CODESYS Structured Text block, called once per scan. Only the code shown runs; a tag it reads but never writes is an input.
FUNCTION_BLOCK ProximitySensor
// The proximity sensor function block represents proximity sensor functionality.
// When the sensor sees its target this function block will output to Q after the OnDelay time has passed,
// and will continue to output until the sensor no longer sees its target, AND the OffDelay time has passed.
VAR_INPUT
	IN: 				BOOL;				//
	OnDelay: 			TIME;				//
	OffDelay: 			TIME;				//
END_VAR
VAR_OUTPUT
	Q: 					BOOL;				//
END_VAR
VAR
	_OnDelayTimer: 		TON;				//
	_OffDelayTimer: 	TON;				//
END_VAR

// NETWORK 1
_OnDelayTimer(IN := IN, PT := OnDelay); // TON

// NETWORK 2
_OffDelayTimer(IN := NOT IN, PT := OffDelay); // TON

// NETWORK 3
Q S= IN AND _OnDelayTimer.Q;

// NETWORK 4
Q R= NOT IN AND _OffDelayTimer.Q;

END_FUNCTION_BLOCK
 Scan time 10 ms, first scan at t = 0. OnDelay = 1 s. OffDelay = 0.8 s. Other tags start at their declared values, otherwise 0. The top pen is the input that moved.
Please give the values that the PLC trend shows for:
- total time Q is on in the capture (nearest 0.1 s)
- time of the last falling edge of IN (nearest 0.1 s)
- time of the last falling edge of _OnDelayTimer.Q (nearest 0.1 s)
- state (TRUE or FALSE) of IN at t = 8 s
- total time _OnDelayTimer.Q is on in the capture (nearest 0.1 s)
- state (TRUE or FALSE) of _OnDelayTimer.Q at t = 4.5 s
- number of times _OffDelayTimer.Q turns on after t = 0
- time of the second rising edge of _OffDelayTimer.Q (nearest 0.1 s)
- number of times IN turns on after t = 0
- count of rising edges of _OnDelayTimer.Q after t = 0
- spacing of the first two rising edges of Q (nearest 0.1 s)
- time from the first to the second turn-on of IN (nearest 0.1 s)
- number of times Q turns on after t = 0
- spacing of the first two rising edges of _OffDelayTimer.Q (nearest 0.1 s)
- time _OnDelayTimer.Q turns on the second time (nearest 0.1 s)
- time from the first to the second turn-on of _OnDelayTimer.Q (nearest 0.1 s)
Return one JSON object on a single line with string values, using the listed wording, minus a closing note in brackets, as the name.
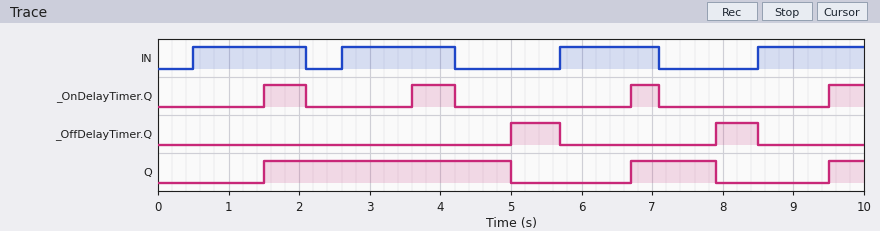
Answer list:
{"total time Q is on in the capture": "5.2 s", "time of the last falling edge of IN": "7.1 s", "time of the last falling edge of _OnDelayTimer.Q": "7.1 s", "state (TRUE or FALSE) of IN at t = 8 s": "FALSE", "total time _OnDelayTimer.Q is on in the capture": "2.1 s", "state (TRUE or FALSE) of _OnDelayTimer.Q at t = 4.5 s": "FALSE", "number of times _OffDelayTimer.Q turns on after t = 0": "2", "time of the second rising edge of _OffDelayTimer.Q": "7.9 s", "number of times IN turns on after t = 0": "4", "count of rising edges of _OnDelayTimer.Q after t = 0": "4", "spacing of the first two rising edges of Q": "5.2 s", "time from the first to the second turn-on of IN": "2.1 s", "number of times Q turns on after t = 0": "3", "spacing of the first two rising edges of _OffDelayTimer.Q": "2.9 s", "time _OnDelayTimer.Q turns on the second time": "3.6 s", "time from the first to the second turn-on of _OnDelayTimer.Q": "2.1 s"}
